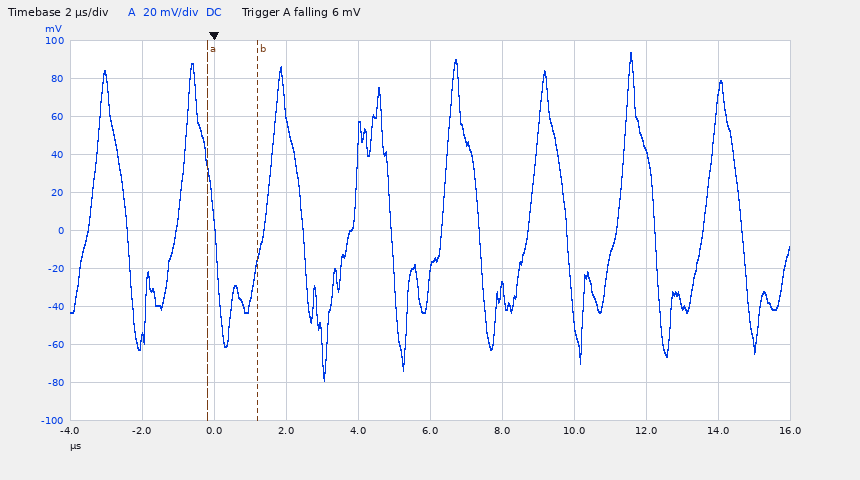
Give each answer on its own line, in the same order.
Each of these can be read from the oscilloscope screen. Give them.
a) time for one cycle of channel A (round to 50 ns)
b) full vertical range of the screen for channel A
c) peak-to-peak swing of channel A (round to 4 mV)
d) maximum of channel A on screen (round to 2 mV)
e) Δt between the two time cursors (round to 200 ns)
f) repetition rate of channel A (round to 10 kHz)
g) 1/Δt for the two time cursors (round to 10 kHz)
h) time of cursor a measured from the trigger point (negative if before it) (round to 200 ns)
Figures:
2.45 µs
200 mV
172 mV
94 mV
1.4 µs
410 kHz
710 kHz
-200 ns
